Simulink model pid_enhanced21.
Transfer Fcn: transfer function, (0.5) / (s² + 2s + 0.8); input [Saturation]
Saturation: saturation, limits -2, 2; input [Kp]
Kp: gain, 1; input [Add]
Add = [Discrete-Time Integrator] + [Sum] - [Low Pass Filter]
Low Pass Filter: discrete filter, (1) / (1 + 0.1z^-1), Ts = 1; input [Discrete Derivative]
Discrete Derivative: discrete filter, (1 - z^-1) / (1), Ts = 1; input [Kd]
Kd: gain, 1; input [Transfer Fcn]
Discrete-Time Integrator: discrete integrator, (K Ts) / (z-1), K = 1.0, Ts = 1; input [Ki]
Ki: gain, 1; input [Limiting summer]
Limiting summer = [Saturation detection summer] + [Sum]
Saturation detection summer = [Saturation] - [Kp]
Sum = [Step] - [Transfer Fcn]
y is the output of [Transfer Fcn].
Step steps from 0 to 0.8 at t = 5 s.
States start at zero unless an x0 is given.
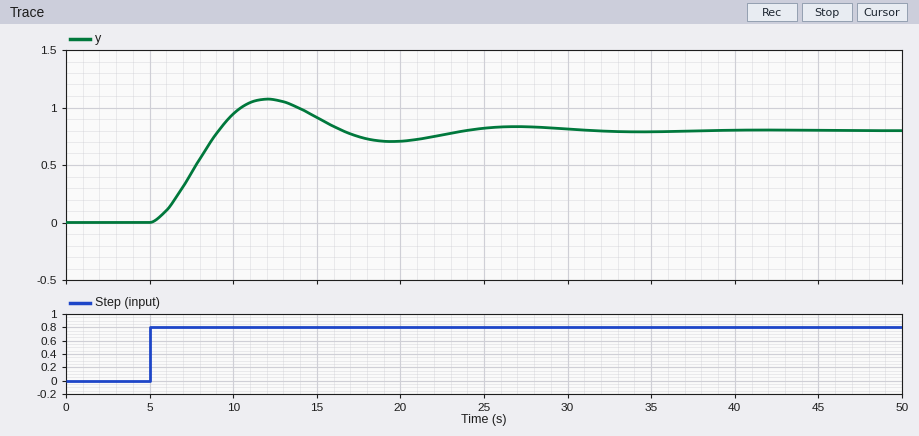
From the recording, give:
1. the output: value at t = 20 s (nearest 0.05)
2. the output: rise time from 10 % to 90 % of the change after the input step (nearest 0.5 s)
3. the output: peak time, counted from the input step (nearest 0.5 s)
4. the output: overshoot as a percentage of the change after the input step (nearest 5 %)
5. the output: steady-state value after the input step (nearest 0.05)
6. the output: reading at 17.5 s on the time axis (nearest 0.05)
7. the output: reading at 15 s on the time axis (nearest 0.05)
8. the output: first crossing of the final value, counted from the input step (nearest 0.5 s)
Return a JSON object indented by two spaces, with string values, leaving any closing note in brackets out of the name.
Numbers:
{
  "the output: value at t = 20 s": "0.70",
  "the output: rise time from 10 % to 90 % of the change after the input step": "3.0 s",
  "the output: peak time, counted from the input step": "7.0 s",
  "the output: overshoot as a percentage of the change after the input step": "35 %",
  "the output: steady-state value after the input step": "0.80",
  "the output: reading at 17.5 s on the time axis": "0.75",
  "the output: reading at 15 s on the time axis": "0.90",
  "the output: first crossing of the final value, counted from the input step": "4.0 s"
}
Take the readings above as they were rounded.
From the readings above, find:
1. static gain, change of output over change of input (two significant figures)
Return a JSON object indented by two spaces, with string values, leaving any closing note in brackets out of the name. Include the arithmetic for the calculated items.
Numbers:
{
  "static gain, change of output over change of input": "(0.8 - 0) / (0.8 - 0) = 1.0"
}
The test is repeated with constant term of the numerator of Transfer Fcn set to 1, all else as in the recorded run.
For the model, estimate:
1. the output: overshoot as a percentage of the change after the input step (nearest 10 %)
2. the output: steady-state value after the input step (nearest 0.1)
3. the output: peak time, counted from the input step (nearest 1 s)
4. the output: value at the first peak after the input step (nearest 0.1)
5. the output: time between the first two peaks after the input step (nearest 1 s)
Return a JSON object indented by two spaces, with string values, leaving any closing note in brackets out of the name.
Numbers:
{
  "the output: overshoot as a percentage of the change after the input step": "50 %",
  "the output: steady-state value after the input step": "0.8",
  "the output: peak time, counted from the input step": "5 s",
  "the output: value at the first peak after the input step": "1.2",
  "the output: time between the first two peaks after the input step": "12 s"
}
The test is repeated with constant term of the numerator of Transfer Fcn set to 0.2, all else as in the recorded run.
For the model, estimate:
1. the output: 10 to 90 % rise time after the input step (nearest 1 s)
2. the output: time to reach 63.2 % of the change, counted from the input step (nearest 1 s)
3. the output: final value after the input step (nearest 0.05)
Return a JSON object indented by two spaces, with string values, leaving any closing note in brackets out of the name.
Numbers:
{
  "the output: 10 to 90 % rise time after the input step": "5 s",
  "the output: time to reach 63.2 % of the change, counted from the input step": "4 s",
  "the output: final value after the input step": "0.50"
}
